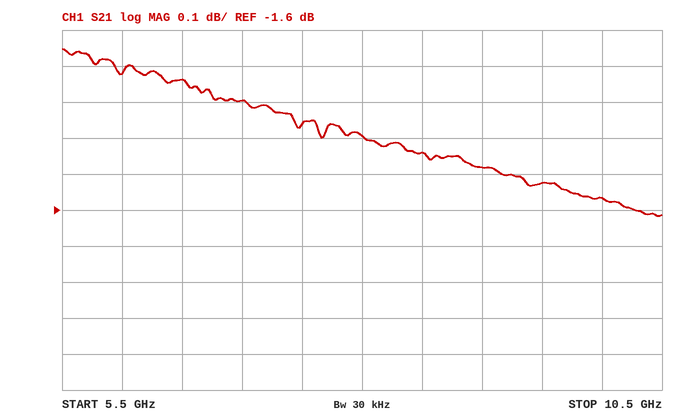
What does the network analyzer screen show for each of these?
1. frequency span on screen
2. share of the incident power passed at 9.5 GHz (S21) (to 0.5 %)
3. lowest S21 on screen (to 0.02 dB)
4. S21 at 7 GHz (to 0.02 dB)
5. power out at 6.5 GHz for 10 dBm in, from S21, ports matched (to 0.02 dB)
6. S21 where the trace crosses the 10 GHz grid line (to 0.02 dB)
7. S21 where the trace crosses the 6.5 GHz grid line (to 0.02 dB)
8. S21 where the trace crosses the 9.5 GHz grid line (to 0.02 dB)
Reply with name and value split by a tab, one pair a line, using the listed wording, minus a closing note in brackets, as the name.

frequency span on screen	5 GHz
share of the incident power passed at 9.5 GHz (S21)	70.5 %
lowest S21 on screen	-1.62 dB
S21 at 7 GHz	-1.30 dB
power out at 6.5 GHz for 10 dBm in, from S21, ports matched	8.76 dBm
S21 where the trace crosses the 10 GHz grid line	-1.56 dB
S21 where the trace crosses the 6.5 GHz grid line	-1.24 dB
S21 where the trace crosses the 9.5 GHz grid line	-1.52 dB
